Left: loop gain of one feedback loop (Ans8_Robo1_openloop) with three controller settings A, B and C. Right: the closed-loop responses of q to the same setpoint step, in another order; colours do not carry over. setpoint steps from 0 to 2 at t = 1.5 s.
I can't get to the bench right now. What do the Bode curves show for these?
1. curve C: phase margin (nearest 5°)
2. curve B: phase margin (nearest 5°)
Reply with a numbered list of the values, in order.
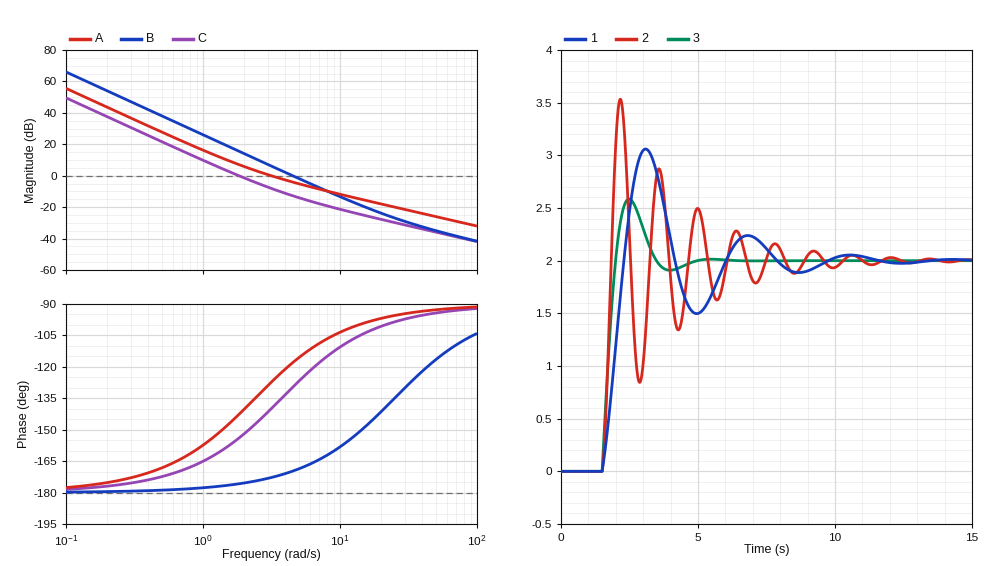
1. 25°
2. 10°
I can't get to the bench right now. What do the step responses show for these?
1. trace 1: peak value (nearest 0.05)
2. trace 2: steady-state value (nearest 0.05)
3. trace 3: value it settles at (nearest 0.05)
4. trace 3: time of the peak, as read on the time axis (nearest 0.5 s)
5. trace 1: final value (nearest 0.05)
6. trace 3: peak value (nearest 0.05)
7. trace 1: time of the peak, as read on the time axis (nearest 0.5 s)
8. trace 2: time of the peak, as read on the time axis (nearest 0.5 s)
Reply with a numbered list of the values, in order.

1. 3.05
2. 2.00
3. 2.00
4. 2.5 s
5. 2.00
6. 2.60
7. 3.0 s
8. 2.0 s
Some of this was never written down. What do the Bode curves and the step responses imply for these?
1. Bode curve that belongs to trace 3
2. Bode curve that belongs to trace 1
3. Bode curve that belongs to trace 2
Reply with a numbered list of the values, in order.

1. A
2. C
3. B
